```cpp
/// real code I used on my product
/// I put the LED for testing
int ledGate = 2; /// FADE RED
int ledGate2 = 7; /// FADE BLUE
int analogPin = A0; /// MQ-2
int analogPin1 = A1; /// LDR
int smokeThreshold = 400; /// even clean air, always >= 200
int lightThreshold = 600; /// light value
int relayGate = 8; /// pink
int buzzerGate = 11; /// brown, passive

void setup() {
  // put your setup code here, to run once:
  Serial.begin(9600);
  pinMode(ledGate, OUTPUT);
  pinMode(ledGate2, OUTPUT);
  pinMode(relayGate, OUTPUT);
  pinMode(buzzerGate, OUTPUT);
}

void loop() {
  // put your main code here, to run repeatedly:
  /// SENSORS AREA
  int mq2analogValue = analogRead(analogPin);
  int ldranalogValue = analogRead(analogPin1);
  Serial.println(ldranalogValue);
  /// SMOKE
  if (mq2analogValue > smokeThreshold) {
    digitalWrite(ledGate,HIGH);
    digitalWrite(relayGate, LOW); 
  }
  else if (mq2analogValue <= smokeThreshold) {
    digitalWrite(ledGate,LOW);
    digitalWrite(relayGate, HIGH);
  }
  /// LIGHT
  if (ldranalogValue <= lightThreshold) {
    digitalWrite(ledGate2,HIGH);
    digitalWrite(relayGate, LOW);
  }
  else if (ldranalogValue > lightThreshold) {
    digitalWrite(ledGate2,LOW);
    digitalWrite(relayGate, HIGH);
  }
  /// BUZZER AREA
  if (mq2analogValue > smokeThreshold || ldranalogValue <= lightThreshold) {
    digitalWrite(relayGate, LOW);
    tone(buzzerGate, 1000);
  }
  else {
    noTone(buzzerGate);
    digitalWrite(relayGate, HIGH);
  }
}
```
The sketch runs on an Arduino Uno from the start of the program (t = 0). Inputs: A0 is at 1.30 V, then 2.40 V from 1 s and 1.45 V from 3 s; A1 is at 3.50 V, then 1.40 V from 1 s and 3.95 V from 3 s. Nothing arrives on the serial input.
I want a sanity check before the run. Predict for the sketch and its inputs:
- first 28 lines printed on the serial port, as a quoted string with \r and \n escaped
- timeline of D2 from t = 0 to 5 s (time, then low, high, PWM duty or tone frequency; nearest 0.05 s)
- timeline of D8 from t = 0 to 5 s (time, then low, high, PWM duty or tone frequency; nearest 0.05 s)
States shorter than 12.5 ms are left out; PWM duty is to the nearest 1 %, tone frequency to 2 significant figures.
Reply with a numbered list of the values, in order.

1. "716\r\n716\r\n716\r\n716\r\n716\r\n716\r\n716\r\n716\r\n716\r\n716\r\n716\r\n716\r\n716\r\n716\r\n716\r\n716\r\n716\r\n716\r\n716\r\n716\r\n716\r\n716\r\n716\r\n716\r\n716\r\n716\r\n716\r\n716\r\n"
2. 0 s low; 1 s high; 3 s low
3. 0 s high; 1 s low; 3 s high
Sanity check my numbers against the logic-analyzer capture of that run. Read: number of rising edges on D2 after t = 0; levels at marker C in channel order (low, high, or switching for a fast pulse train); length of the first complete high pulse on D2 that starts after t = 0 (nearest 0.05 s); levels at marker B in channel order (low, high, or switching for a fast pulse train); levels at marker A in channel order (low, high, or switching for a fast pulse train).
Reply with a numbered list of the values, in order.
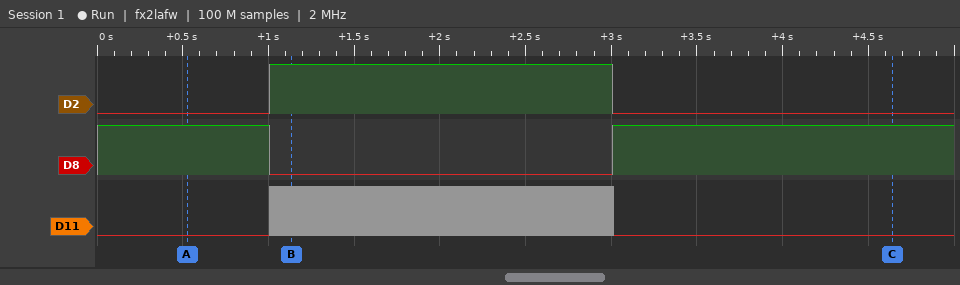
1. 1
2. D2 low, D8 high, D11 low
3. 2.00 s
4. D2 high, D8 low, D11 switching
5. D2 low, D8 high, D11 low
